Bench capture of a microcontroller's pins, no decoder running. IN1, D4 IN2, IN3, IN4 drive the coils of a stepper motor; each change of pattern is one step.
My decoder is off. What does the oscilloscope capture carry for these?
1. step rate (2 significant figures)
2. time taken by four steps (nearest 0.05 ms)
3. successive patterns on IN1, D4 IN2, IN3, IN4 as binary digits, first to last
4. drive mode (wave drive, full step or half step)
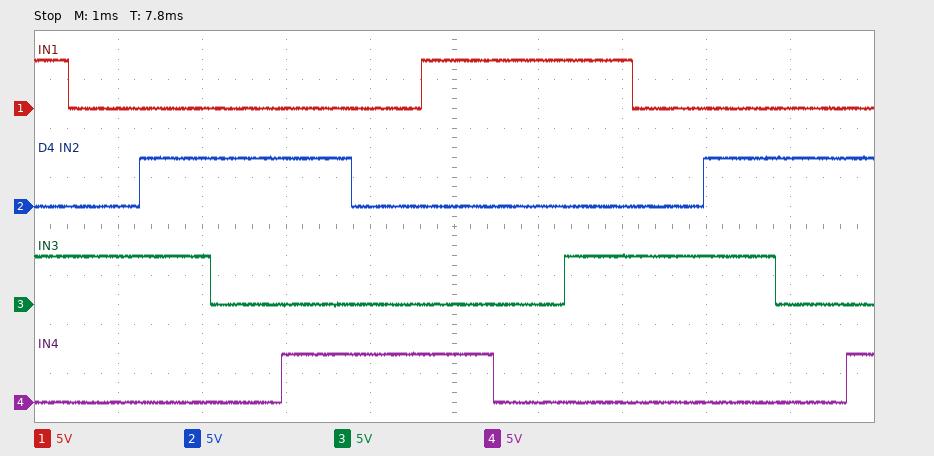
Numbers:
1200 steps/s
3.35 ms
1010 0010 0110 0100 0101 0001 1001 1000 1010 0010 0110 0100 0101
half step
